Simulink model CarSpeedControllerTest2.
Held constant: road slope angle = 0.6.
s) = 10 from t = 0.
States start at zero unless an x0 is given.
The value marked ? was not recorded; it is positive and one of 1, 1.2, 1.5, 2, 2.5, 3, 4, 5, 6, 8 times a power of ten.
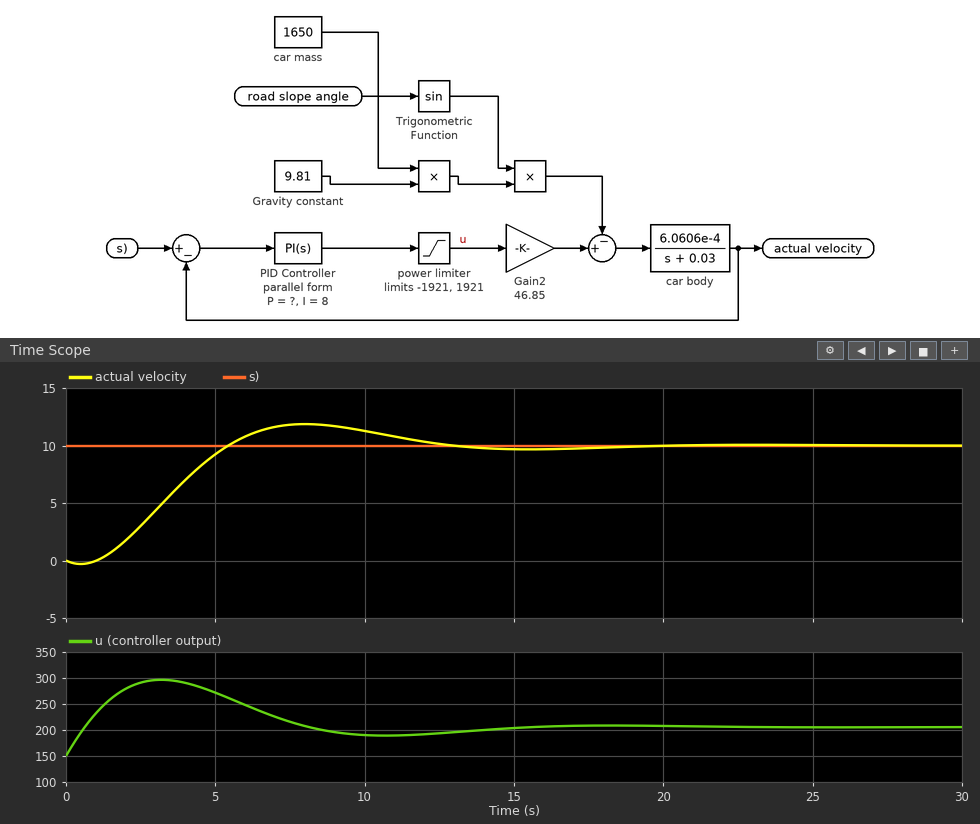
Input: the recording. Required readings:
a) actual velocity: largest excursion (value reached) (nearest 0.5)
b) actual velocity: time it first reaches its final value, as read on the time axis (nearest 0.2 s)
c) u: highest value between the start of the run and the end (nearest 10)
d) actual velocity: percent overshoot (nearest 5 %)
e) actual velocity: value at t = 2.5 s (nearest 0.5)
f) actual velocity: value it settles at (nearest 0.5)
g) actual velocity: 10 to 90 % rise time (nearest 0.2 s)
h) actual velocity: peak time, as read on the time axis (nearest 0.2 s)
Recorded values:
12.0
5.4 s
300
20 %
3.0
10.0
3.2 s
8.0 s
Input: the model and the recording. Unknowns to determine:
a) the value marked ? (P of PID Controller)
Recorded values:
15
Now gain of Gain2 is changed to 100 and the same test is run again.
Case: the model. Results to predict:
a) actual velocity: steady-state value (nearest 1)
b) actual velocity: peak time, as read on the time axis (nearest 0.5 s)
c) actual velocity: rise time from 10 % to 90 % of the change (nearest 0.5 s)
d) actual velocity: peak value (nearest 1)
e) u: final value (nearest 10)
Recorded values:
10
5.0 s
2.5 s
11
100
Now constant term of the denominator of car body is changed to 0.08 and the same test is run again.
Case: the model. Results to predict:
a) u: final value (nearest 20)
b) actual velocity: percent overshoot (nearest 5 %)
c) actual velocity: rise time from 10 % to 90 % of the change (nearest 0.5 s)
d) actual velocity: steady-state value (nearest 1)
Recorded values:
220
15 %
3.5 s
10
